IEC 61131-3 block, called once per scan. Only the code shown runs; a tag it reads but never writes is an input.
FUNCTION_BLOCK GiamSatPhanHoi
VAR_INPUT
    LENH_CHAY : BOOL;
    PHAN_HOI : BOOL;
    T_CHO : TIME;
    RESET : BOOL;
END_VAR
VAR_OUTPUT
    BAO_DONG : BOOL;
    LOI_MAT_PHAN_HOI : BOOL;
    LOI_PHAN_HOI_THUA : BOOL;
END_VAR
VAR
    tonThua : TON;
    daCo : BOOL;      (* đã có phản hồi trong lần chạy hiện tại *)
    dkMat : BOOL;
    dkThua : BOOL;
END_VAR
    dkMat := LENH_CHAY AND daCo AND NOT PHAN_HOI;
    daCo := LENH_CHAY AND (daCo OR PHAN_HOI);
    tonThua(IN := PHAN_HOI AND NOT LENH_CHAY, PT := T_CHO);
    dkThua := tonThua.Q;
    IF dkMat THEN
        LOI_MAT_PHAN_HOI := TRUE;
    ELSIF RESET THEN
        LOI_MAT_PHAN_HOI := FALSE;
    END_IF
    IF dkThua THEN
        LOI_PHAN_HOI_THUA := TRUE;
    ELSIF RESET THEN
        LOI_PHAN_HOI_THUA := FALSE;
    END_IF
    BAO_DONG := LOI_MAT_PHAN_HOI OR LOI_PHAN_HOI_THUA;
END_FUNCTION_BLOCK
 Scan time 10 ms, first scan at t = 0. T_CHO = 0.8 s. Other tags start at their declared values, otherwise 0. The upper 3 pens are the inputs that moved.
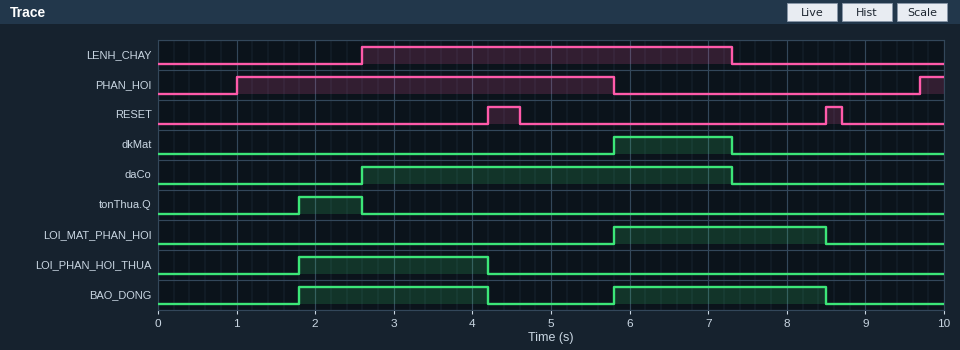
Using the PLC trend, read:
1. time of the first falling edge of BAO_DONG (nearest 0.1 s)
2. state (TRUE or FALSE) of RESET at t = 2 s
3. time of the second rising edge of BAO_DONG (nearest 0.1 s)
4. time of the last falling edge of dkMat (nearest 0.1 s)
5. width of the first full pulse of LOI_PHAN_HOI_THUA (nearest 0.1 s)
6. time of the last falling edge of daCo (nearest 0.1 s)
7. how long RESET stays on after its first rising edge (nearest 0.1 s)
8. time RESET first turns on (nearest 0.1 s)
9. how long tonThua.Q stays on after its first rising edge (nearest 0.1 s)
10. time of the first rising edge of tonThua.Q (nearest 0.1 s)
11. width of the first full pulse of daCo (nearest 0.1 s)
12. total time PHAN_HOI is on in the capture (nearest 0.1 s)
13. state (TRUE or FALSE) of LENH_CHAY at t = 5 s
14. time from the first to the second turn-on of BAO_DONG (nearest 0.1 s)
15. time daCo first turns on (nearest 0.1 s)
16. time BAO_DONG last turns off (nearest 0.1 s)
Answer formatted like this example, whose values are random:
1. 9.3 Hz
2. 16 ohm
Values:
1. 4.2 s
2. FALSE
3. 5.8 s
4. 7.3 s
5. 2.4 s
6. 7.3 s
7. 0.4 s
8. 4.2 s
9. 0.8 s
10. 1.8 s
11. 4.7 s
12. 5.1 s
13. TRUE
14. 4.0 s
15. 2.6 s
16. 8.5 s
